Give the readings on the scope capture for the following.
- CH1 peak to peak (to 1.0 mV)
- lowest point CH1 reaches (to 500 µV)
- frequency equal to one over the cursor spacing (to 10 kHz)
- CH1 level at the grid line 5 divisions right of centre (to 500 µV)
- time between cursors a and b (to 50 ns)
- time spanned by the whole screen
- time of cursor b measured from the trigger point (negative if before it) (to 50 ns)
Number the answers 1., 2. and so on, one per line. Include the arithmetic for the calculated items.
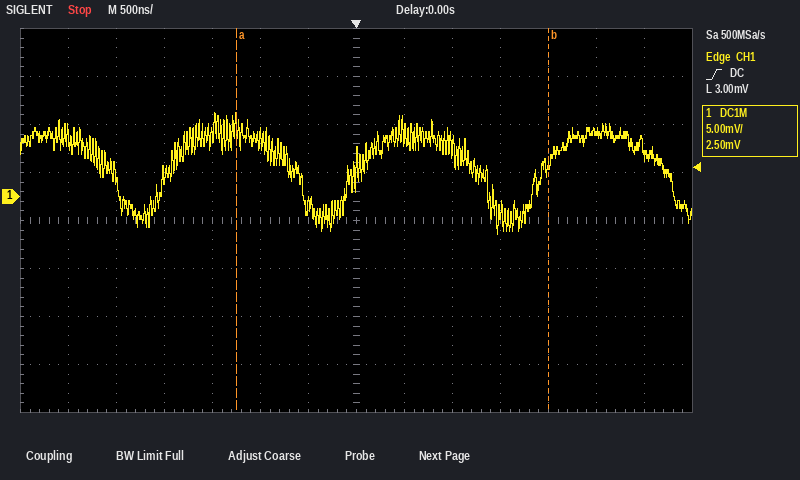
1. 13.0 mV
2. -4.0 mV
3. 1 / 3.25 µs ≈ 310 kHz
4. 7.0 mV
5. 3.25 µs
6. 7 µs
7. +2.00 µs
